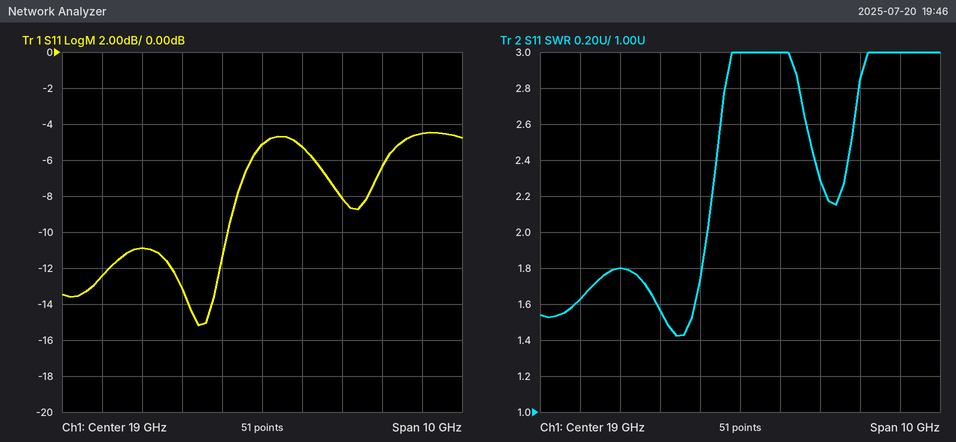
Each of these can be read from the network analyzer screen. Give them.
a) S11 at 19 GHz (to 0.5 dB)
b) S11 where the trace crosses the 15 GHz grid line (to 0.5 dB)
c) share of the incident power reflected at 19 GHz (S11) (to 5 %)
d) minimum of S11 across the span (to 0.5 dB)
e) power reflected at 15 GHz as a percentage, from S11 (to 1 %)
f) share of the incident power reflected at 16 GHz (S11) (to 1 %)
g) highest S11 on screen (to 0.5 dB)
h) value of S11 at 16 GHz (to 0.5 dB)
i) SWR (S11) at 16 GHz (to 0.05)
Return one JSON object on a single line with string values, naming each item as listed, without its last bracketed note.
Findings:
{"S11 at 19 GHz": "-5.0 dB", "S11 where the trace crosses the 15 GHz grid line": "-12.5 dB", "share of the incident power reflected at 19 GHz (S11)": "30 %", "minimum of S11 across the span": "-15.0 dB", "power reflected at 15 GHz as a percentage, from S11": "6 %", "share of the incident power reflected at 16 GHz (S11)": "8 %", "highest S11 on screen": "-4.5 dB", "value of S11 at 16 GHz": "-11.0 dB", "SWR (S11) at 16 GHz": "1.80"}
